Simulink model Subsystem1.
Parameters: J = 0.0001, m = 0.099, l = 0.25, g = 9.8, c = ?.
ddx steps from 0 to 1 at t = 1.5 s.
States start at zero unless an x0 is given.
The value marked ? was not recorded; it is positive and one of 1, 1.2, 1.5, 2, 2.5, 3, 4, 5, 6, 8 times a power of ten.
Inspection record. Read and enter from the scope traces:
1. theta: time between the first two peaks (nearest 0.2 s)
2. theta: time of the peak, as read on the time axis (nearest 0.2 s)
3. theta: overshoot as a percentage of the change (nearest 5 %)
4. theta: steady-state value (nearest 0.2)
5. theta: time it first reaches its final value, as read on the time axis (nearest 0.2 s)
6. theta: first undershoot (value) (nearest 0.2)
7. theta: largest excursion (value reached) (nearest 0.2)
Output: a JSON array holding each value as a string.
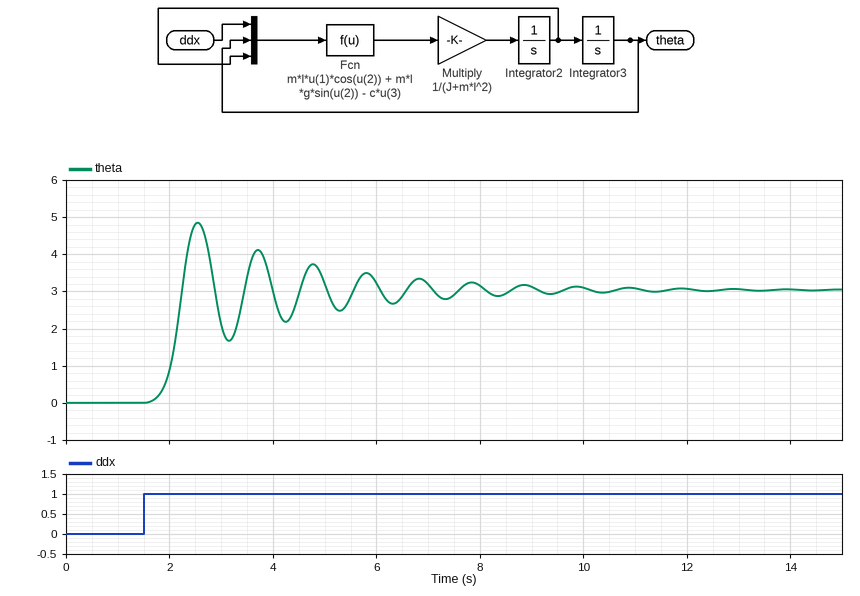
["1.2 s", "2.6 s", "60 %", "3.0", "2.2 s", "1.6", "4.8"]
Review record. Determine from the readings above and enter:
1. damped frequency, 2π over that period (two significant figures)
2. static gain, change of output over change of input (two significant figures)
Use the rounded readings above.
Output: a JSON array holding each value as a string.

["5.2 rad/s", "3.0"]
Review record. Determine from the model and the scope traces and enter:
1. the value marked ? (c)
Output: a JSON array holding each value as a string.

["0.005"]
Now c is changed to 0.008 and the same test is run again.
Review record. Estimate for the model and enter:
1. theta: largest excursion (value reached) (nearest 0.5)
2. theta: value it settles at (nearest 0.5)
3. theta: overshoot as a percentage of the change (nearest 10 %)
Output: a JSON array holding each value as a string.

["4.5", "3.0", "50 %"]
